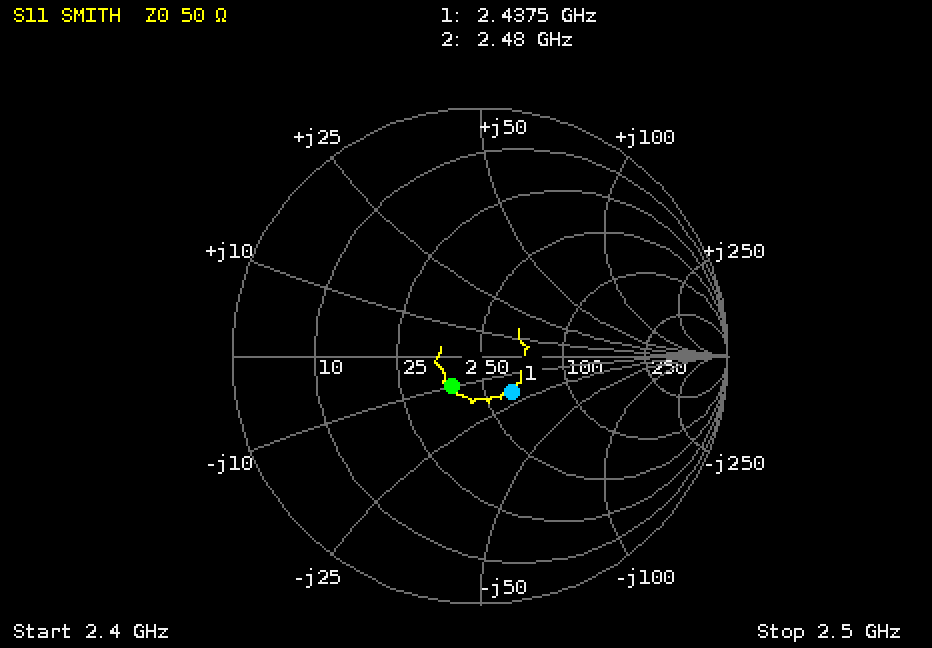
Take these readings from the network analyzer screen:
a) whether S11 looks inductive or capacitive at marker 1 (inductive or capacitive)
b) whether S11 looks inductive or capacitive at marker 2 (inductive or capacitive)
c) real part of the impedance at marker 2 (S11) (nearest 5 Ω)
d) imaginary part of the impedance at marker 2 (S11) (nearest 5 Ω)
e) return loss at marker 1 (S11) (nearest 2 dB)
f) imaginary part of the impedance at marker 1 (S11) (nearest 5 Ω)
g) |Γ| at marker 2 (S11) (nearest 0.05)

capacitive
capacitive
40 Ω
-10 Ω
14 dB
-20 Ω
0.15
